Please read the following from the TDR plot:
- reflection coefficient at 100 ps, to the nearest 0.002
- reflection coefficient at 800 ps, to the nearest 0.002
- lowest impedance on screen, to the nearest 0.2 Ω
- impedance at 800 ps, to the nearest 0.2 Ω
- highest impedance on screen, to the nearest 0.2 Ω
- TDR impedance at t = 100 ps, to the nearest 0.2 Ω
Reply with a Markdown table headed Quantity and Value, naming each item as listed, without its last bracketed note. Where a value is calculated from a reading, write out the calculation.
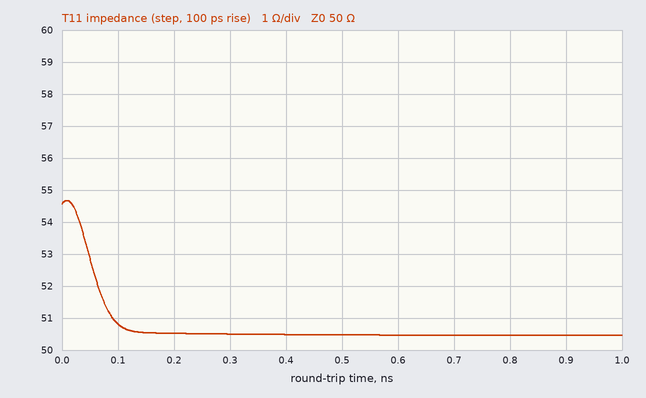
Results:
| Quantity | Value |
|---|---|
| reflection coefficient at 100 ps, to the nearest 0.002 | (50.8 − 50)/(50.8 + 50) ≈ +0.008 |
| reflection coefficient at 800 ps, to the nearest 0.002 | (50.4 − 50)/(50.4 + 50) ≈ +0.004 |
| lowest impedance on screen, to the nearest 0.2 Ω | 50.4 Ω |
| impedance at 800 ps, to the nearest 0.2 Ω | 50.4 Ω |
| highest impedance on screen, to the nearest 0.2 Ω | 54.6 Ω |
| TDR impedance at t = 100 ps, to the nearest 0.2 Ω | 50.8 Ω |
